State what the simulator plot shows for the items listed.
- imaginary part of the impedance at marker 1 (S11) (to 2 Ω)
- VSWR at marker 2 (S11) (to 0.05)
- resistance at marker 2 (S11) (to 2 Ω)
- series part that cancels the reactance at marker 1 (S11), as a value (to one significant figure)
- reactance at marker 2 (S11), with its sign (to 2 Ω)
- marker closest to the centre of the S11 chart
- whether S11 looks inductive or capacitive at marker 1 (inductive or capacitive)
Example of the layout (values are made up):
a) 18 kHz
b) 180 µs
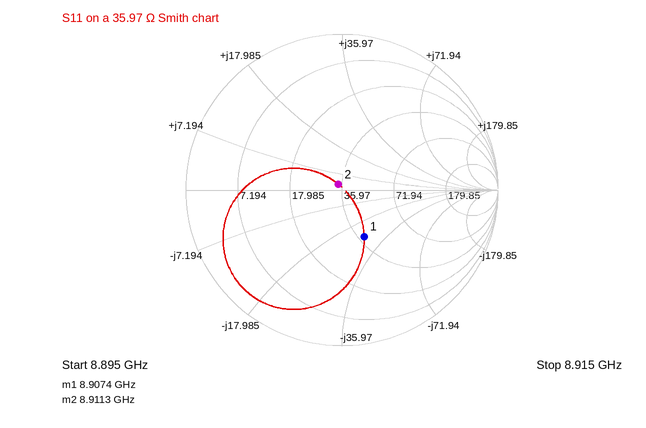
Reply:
a) -26 Ω
b) 1.10
c) 34 Ω
d) 500 pH
e) +2 Ω
f) marker 2
g) capacitive
